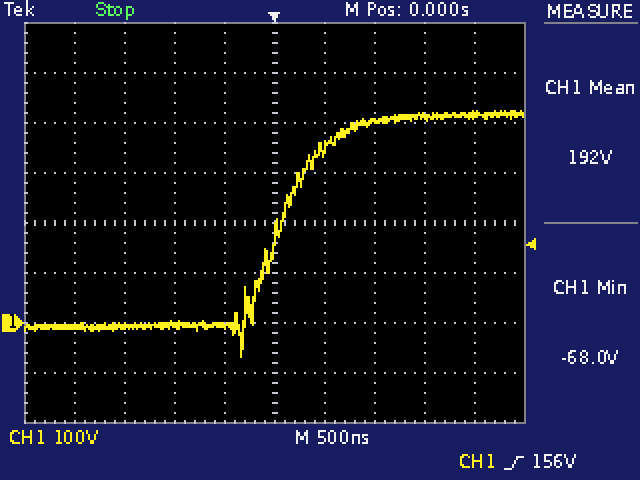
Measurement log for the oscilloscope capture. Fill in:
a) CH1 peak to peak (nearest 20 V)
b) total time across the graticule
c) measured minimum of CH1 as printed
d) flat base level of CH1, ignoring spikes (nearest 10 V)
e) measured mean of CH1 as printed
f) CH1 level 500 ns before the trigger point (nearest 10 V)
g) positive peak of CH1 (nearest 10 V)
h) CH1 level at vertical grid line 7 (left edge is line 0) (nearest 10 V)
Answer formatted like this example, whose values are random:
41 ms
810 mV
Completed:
500 V
5 µs
-68.0 V
-10 V
192 V
-10 V
420 V
400 V
